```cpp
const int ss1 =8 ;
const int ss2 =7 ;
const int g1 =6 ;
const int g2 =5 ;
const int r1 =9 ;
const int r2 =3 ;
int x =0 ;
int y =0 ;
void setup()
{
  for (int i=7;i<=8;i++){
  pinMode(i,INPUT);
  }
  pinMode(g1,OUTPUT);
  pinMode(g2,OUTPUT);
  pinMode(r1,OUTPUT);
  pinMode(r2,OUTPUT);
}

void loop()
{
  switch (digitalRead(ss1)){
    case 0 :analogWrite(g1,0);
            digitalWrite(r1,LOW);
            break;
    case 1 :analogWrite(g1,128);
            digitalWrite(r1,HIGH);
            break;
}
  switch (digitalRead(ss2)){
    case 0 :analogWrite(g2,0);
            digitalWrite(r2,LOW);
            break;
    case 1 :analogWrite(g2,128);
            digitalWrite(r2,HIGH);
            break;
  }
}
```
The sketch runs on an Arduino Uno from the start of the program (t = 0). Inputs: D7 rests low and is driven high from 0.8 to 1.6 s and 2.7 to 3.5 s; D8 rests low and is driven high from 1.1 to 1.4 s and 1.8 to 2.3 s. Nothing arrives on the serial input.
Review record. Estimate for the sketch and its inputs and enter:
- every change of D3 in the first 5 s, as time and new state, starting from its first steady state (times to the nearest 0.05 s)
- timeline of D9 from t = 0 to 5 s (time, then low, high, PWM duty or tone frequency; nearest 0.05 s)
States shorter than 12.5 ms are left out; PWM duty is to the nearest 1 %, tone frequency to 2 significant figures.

0 s low; 0.8 s high; 1.6 s low; 2.7 s high; 3.5 s low
0 s low; 1.1 s high; 1.4 s low; 1.8 s high; 2.3 s low
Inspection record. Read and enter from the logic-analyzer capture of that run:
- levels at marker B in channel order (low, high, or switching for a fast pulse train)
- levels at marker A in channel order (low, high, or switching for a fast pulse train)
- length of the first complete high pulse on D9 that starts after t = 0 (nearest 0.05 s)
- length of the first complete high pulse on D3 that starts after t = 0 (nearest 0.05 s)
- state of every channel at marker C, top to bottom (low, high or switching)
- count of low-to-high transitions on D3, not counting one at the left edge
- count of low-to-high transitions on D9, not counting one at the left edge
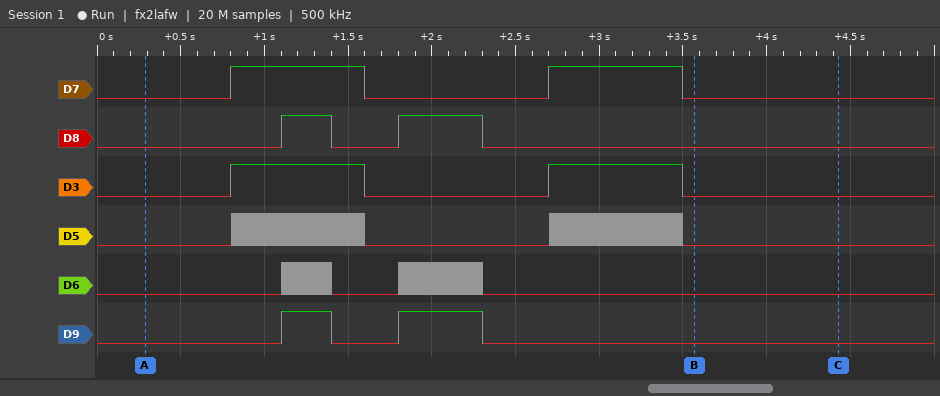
D7 low, D8 low, D3 low, D5 low, D6 low, D9 low
D7 low, D8 low, D3 low, D5 low, D6 low, D9 low
0.30 s
0.80 s
D7 low, D8 low, D3 low, D5 low, D6 low, D9 low
2
2
